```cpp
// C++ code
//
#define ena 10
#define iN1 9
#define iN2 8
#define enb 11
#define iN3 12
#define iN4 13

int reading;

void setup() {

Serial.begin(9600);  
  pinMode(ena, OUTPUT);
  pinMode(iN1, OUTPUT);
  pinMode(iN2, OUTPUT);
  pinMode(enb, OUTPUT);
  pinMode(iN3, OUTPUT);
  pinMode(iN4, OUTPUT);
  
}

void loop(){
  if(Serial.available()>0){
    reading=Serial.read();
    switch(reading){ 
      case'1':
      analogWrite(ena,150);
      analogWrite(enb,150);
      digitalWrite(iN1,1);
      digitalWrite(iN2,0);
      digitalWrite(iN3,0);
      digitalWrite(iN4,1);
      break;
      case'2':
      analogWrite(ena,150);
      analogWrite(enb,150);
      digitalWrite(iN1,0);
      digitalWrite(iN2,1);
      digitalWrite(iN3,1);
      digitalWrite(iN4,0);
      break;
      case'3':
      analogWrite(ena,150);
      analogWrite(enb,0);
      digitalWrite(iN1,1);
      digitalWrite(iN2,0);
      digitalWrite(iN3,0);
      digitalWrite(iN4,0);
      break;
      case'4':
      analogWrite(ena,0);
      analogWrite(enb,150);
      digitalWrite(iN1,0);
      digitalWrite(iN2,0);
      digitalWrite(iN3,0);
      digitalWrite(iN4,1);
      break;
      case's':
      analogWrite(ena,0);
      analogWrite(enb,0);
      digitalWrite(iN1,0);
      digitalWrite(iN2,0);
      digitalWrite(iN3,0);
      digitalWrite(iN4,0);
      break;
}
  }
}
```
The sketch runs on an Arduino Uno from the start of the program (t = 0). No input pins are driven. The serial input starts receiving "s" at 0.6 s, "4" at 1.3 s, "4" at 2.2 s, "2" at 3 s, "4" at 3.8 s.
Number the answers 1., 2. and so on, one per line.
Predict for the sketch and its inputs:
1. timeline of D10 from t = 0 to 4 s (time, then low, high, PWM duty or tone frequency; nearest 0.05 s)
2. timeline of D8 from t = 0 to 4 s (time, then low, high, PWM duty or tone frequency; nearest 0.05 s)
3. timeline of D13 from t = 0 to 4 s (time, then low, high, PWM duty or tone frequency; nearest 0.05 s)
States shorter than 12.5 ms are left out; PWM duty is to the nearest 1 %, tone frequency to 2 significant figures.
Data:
1. 0 s low; 3 s PWM 59 %; 3.8 s low
2. 0 s low; 3 s high; 3.8 s low
3. 0 s low; 1.3 s high; 3 s low; 3.8 s high
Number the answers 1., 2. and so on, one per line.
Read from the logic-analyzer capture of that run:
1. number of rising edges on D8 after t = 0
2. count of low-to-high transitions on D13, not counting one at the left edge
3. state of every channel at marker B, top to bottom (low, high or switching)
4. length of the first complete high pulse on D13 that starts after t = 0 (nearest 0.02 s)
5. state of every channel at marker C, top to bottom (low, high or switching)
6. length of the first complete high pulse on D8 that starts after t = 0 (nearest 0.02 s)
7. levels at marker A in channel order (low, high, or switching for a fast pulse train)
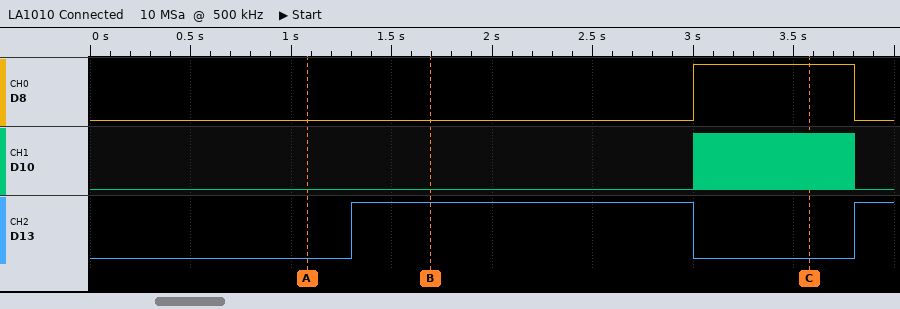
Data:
1. 1
2. 2
3. D8 low, D10 low, D13 high
4. 1.70 s
5. D8 high, D10 switching, D13 low
6. 0.80 s
7. D8 low, D10 low, D13 low
